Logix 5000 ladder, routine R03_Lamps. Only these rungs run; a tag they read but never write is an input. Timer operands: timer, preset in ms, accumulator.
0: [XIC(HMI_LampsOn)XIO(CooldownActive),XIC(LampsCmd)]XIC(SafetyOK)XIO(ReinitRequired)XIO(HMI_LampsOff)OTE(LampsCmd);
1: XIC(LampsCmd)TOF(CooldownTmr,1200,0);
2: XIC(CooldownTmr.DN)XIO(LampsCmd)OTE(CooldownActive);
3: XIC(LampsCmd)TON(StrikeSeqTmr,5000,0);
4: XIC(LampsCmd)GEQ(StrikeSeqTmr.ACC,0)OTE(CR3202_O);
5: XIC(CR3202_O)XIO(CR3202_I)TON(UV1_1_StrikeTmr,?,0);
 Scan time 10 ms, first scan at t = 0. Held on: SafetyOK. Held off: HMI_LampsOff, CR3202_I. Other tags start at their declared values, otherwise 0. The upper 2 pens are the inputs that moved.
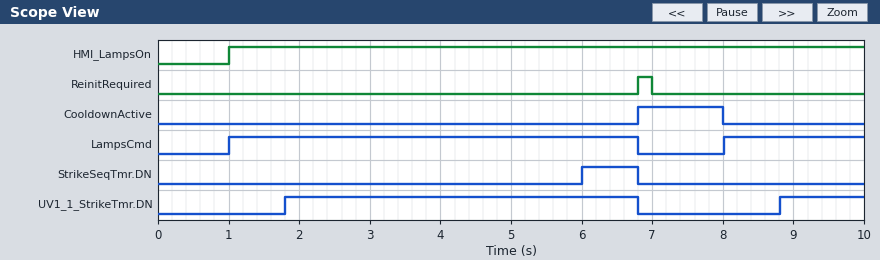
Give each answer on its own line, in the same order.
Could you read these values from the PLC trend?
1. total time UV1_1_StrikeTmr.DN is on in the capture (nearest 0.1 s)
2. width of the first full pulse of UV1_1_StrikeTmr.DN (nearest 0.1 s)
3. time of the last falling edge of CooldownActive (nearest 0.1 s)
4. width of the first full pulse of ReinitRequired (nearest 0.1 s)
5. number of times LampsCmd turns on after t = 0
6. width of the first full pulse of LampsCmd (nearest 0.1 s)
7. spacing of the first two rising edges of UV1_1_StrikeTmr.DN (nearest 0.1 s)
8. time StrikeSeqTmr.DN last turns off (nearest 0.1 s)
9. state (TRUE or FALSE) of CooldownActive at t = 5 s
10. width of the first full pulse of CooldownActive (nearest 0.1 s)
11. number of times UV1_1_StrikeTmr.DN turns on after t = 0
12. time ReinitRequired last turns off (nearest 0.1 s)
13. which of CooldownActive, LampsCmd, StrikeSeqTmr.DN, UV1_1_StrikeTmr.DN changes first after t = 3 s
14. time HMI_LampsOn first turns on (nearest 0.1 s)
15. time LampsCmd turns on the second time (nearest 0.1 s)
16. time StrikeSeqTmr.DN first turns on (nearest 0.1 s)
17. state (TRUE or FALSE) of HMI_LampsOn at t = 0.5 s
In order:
6.2 s
5.0 s
8.0 s
0.2 s
2
5.8 s
7.0 s
6.8 s
FALSE
1.2 s
2
7.0 s
StrikeSeqTmr.DN
1.0 s
8.0 s
6.0 s
FALSE
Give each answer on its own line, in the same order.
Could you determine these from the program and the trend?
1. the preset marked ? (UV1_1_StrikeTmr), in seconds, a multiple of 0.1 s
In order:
0.8 s
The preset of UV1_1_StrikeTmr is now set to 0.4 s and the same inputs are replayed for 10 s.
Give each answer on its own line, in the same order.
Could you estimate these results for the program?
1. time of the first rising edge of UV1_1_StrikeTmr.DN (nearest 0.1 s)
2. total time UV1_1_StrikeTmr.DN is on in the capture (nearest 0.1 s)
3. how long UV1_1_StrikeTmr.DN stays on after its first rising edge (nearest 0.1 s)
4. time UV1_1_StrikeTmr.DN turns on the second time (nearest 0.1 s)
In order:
1.4 s
7.0 s
5.4 s
8.4 s
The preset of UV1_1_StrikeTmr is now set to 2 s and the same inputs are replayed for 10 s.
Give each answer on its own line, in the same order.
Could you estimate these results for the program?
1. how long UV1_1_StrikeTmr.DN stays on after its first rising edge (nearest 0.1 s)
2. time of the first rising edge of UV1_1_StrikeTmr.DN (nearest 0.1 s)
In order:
3.8 s
3.0 s
